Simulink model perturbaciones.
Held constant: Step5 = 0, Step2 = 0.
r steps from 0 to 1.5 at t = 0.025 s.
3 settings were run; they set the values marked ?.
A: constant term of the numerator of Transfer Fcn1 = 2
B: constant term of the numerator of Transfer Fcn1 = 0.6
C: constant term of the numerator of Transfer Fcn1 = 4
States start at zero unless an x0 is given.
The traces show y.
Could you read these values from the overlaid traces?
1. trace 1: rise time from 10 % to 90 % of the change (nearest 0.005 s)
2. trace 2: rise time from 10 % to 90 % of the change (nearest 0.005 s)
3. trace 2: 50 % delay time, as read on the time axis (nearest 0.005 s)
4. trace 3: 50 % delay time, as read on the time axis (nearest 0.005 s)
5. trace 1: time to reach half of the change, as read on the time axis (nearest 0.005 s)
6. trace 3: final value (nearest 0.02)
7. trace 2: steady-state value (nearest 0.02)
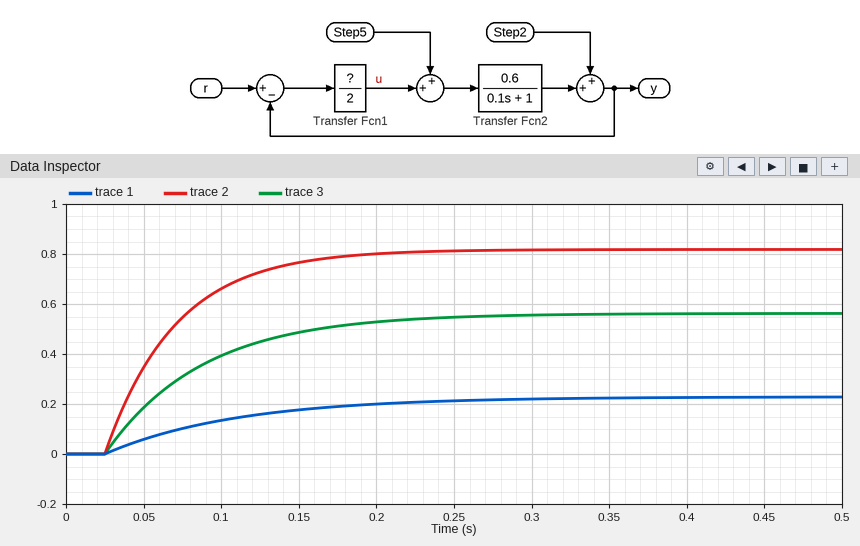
0.185 s
0.100 s
0.055 s
0.070 s
0.085 s
0.56
0.82
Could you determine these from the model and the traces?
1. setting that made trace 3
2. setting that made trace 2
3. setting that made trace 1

A
C
B
